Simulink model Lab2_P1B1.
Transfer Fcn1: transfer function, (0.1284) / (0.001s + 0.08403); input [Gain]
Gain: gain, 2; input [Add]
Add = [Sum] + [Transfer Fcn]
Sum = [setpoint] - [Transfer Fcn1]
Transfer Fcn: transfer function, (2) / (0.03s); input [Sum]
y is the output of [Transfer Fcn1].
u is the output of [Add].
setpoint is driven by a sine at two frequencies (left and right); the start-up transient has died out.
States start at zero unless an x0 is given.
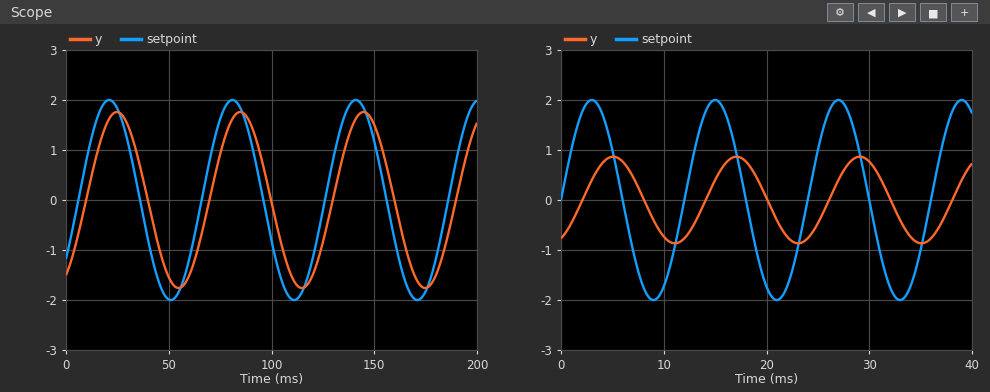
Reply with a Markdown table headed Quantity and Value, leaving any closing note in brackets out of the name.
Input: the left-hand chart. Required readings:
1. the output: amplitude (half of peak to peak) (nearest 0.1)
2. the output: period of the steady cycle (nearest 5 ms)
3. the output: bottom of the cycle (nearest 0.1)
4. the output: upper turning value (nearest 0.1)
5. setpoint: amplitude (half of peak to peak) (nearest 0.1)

| Quantity | Value |
|---|---|
| the output: amplitude (half of peak to peak) | 1.8 |
| the output: period of the steady cycle | 60 ms |
| the output: bottom of the cycle | -1.8 |
| the output: upper turning value | 1.8 |
| setpoint: amplitude (half of peak to peak) | 2.0 |
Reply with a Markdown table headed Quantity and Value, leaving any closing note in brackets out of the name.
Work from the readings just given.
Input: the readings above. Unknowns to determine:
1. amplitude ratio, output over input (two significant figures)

| Quantity | Value |
|---|---|
| amplitude ratio, output over input | 0.90 |
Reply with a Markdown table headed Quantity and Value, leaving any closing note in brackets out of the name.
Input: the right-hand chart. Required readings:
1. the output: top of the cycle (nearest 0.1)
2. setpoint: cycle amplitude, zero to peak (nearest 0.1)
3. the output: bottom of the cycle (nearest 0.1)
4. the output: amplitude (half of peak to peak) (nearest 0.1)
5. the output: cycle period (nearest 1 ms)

| Quantity | Value |
|---|---|
| the output: top of the cycle | 0.9 |
| setpoint: cycle amplitude, zero to peak | 2.0 |
| the output: bottom of the cycle | -0.9 |
| the output: amplitude (half of peak to peak) | 0.9 |
| the output: cycle period | 12 ms |
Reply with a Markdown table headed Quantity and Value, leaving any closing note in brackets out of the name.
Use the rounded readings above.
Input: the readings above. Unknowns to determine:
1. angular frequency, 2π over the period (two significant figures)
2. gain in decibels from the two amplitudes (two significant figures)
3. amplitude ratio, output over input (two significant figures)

| Quantity | Value |
|---|---|
| angular frequency, 2π over the period | 0.52 rad/ms |
| gain in decibels from the two amplitudes | -6.9 dB |
| amplitude ratio, output over input | 0.45 |
